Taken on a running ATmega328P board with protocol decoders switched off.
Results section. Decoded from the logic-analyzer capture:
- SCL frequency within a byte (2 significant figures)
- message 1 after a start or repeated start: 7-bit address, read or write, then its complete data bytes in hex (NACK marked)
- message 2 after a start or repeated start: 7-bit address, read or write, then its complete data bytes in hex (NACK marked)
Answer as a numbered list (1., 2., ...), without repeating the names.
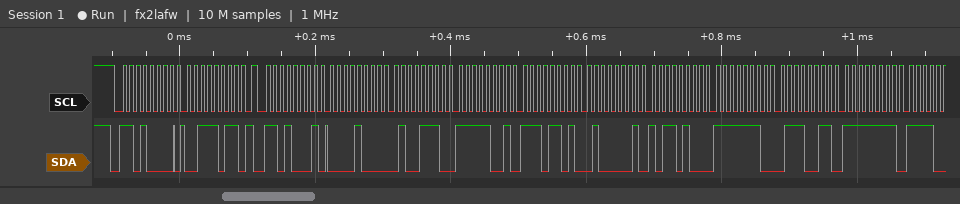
1. 100 kHz
2. 0x68 write: 3B
3. 0x68 read: 08 4E F9 ED 41 B4 FE 73 FF
